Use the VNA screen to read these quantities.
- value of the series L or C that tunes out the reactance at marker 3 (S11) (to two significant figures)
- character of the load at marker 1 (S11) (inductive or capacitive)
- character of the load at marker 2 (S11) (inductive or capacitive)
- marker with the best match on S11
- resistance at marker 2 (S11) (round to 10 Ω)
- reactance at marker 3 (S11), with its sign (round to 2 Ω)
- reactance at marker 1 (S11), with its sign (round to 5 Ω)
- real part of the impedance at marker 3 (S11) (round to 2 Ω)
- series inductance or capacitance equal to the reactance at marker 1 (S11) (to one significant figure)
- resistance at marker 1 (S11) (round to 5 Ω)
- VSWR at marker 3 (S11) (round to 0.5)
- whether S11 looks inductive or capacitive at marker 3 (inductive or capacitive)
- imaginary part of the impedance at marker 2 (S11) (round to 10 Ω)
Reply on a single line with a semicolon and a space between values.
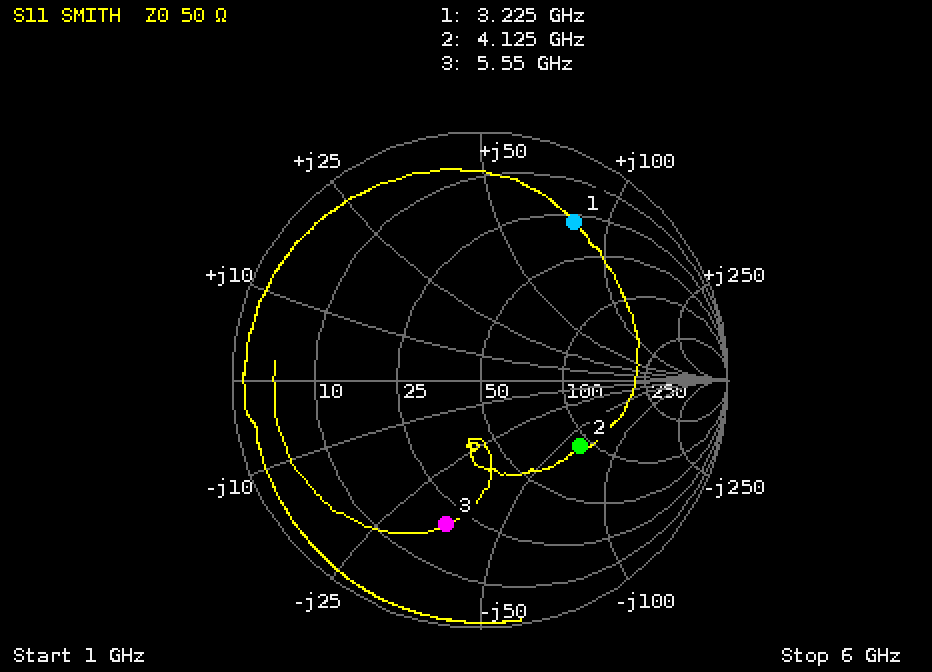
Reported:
1.0 nH; inductive; capacitive; marker 2; 90 Ω; -36 Ω; +80 Ω; 20 Ω; 4 nH; 30 Ω; 4.0; capacitive; -60 Ω
